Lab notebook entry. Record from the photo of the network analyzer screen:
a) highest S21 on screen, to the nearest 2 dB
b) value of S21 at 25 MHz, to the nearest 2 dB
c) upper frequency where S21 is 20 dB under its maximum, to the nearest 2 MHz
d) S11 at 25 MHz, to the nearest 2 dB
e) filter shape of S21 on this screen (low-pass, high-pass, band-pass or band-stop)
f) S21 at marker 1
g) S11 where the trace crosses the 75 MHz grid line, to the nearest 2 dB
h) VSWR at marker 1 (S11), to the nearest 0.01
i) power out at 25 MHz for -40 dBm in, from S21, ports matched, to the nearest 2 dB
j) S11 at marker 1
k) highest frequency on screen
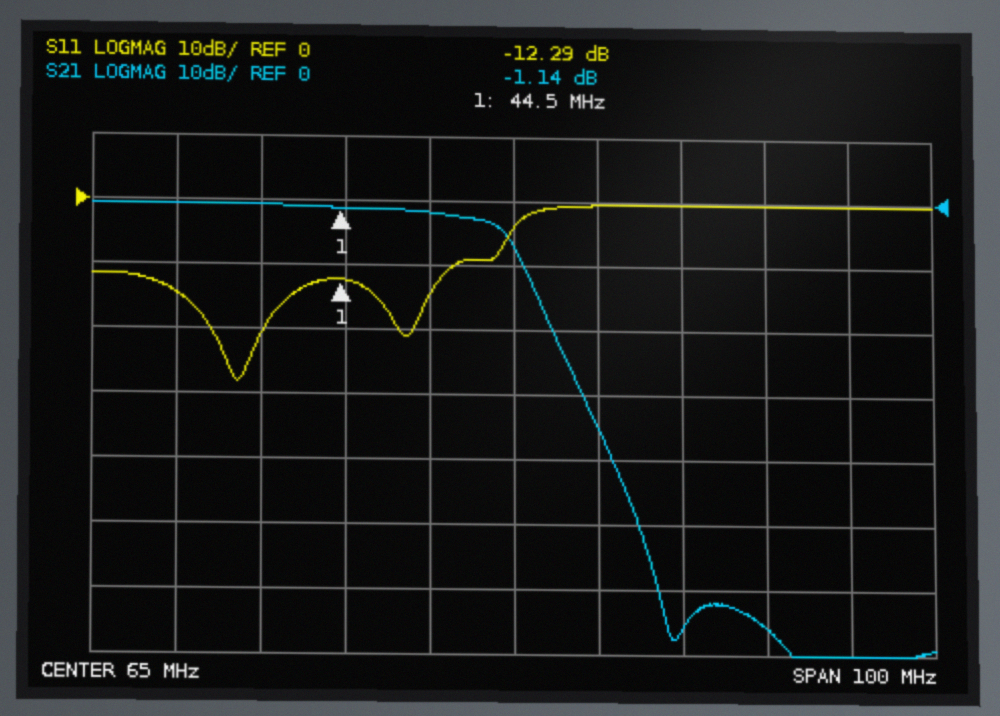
0 dB
0 dB
70 MHz
-14 dB
low-pass
-1.14 dB
0 dB
1.64
-40 dBm
-12.29 dB
115 MHz
